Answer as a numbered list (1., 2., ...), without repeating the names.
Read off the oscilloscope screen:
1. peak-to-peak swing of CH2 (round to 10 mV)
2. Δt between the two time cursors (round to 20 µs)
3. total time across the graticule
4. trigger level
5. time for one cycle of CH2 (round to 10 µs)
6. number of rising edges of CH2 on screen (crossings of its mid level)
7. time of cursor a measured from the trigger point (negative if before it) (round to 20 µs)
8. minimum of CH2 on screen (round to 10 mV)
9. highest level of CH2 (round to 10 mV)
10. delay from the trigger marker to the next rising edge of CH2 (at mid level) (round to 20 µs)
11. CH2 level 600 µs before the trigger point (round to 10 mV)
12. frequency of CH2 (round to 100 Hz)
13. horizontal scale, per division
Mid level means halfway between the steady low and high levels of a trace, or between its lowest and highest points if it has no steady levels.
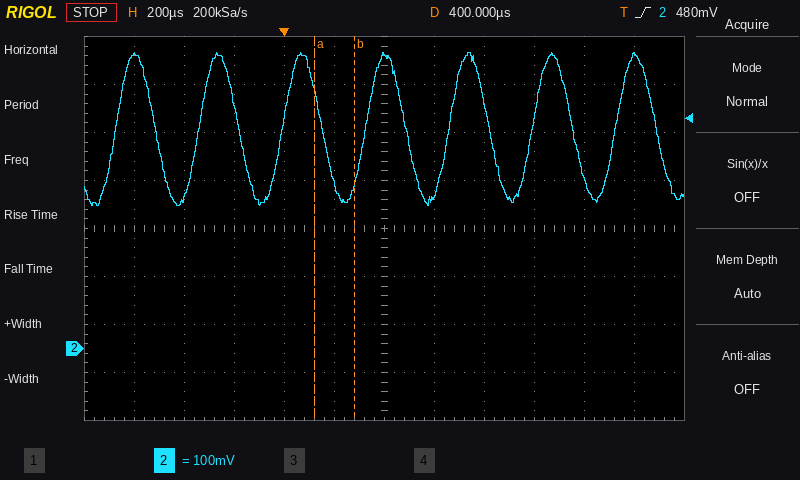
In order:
1. 320 mV
2. 160 µs
3. 2.4 ms
4. 480 mV
5. 330 µs
6. 7
7. +120 µs
8. 300 mV
9. 620 mV
10. 320 µs
11. 610 mV
12. 3.0 kHz
13. 200 µs
